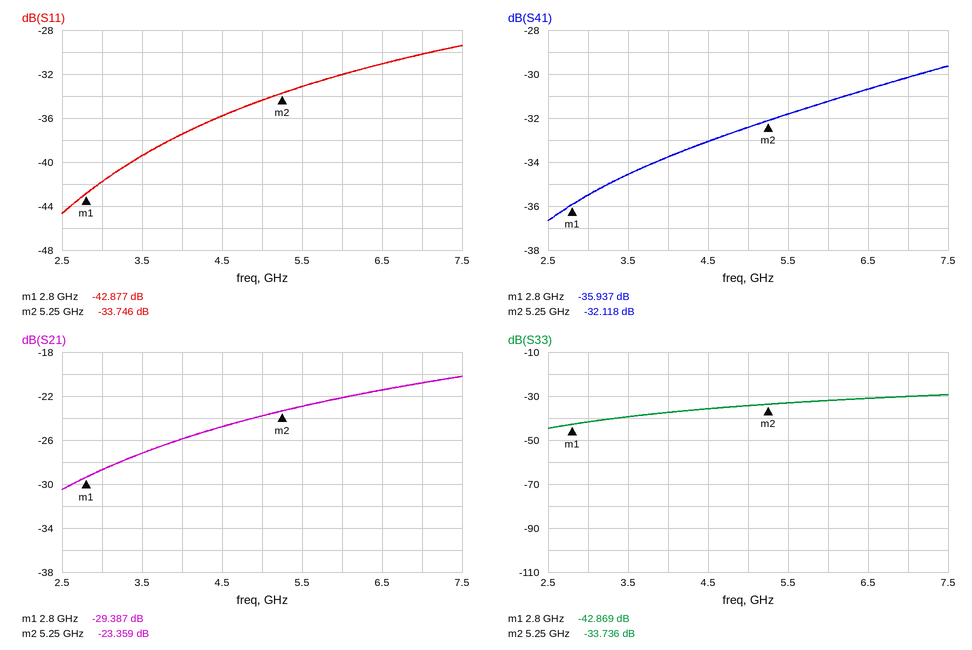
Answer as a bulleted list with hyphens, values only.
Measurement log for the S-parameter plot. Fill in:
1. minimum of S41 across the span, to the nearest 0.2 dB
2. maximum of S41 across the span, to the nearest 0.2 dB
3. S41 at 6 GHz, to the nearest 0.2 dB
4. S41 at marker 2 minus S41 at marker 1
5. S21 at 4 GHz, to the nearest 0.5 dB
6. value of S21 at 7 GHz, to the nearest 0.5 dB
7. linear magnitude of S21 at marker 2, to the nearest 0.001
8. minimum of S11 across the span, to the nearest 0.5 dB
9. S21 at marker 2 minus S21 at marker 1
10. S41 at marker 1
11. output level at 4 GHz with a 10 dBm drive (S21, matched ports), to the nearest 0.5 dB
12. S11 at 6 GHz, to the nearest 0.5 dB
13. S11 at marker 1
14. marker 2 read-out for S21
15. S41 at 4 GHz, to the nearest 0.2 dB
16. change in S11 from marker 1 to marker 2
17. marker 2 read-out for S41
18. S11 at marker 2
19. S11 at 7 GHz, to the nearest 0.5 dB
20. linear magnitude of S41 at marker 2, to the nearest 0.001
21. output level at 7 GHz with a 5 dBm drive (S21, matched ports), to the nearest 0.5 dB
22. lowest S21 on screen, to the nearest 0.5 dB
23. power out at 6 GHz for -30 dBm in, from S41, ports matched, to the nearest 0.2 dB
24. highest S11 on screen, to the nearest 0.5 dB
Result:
- -36.6 dB
- -29.6 dB
- -31.2 dB
- 3.819 dB
- -26.0 dB
- -21.0 dB
- 0.068
- -44.5 dB
- 6.028 dB
- -35.937 dB
- -16.0 dBm
- -32.0 dB
- -42.877 dB
- -23.359 dB
- -33.8 dB
- 9.131 dB
- -32.118 dB
- -33.746 dB
- -30.0 dB
- 0.025
- -16.0 dBm
- -30.5 dB
- -61.2 dBm
- -29.5 dB
